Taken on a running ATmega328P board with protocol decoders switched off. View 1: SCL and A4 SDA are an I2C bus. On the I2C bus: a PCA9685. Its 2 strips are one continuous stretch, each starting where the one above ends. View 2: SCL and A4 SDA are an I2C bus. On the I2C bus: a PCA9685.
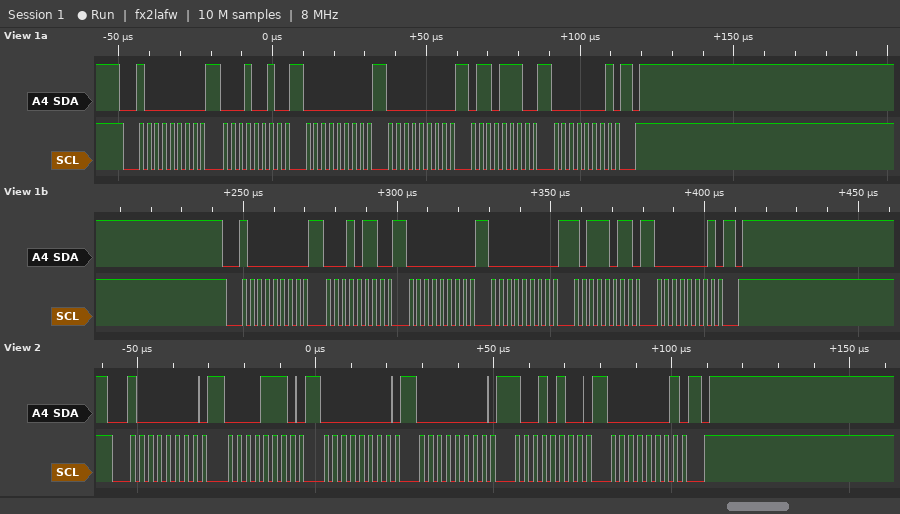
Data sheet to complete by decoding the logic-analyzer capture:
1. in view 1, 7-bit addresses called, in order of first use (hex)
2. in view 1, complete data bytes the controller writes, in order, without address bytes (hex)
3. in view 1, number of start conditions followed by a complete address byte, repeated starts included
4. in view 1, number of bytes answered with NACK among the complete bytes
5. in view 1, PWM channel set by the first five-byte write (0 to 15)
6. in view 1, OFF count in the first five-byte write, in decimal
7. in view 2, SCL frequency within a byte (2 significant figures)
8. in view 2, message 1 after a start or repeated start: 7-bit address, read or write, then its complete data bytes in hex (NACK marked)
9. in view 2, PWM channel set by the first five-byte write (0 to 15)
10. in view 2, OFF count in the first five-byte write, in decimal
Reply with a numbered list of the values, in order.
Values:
1. 0x40
2. 12 00 00 6E 01 16 00 00 BB 01
3. 2
4. 0
5. 3
6. 366
7. 400 kHz
8. 0x40 write: 0E 00 00 94 01
9. 2
10. 404
